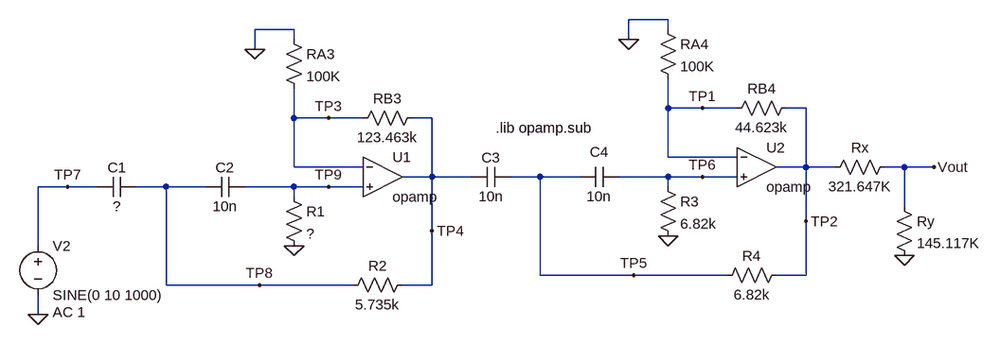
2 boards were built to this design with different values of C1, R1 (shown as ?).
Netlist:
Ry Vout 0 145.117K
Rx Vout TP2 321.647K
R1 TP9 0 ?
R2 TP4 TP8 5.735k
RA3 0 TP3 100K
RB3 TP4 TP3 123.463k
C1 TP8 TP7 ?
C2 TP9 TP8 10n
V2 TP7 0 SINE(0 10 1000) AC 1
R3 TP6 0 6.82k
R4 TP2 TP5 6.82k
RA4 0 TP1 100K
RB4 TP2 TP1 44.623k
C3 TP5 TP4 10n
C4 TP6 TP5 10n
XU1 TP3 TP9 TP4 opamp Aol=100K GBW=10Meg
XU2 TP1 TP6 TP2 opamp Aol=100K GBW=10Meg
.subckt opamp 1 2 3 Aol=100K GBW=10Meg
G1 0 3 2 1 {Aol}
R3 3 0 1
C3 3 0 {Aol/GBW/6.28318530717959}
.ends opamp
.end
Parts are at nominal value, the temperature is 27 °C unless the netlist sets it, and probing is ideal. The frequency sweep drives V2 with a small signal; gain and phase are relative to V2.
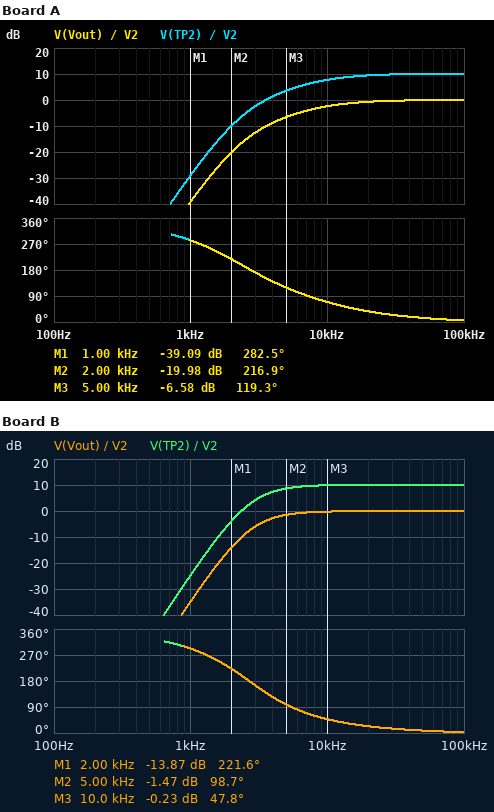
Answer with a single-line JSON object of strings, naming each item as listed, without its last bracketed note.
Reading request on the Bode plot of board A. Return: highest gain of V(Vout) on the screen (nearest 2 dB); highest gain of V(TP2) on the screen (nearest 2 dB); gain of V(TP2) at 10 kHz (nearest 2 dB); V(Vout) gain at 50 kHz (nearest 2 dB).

{"highest gain of V(Vout) on the screen": "0 dB", "highest gain of V(TP2) on the screen": "10 dB", "gain of V(TP2) at 10 kHz": "8 dB", "V(Vout) gain at 50 kHz": "0 dB"}
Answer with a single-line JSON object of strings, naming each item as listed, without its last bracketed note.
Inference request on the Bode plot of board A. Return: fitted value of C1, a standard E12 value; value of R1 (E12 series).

{"fitted value of C1, a standard E12 value": "15 nF", "value of R1": "2.2 kΩ"}
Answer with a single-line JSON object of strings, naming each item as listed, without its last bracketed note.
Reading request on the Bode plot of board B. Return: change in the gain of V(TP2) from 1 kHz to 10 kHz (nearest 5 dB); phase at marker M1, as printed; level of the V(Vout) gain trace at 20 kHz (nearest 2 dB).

{"change in the gain of V(TP2) from 1 kHz to 10 kHz": "35 dB", "phase at marker M1, as printed": "221.6 deg", "level of the V(Vout) gain trace at 20 kHz": "0 dB"}
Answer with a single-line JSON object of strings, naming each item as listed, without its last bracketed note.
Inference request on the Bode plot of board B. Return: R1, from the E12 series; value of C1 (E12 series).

{"R1, from the E12 series": "3.9 kΩ", "value of C1": "12 nF"}
